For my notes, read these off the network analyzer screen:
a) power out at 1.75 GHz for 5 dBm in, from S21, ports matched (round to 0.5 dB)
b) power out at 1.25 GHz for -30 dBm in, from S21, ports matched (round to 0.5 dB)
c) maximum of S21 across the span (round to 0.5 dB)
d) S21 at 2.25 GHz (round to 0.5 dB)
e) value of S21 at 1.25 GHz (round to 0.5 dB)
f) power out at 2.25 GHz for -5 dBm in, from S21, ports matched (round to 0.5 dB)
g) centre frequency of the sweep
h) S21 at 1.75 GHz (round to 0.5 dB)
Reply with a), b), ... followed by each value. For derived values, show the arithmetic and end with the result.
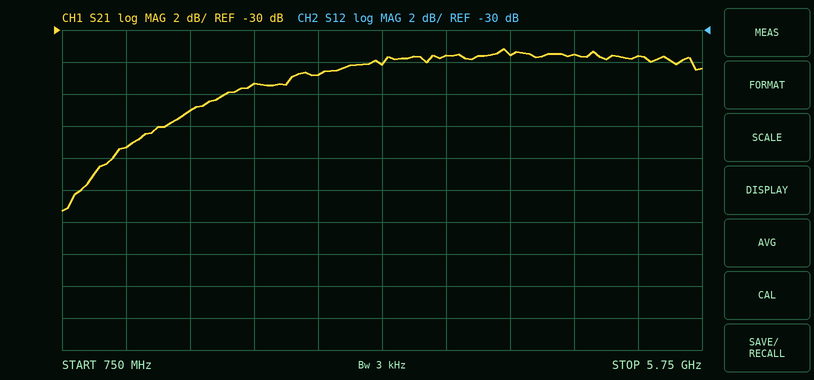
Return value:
a) 5 dBm + (-35.0 dB) = -30.0 dBm
b) -30 dBm + (-37.5 dB) = -67.5 dBm
c) -31.0 dB
d) -33.5 dB
e) -37.5 dB
f) -5 dBm + (-33.5 dB) = -38.5 dBm
g) 3.25 GHz
h) -35.0 dB
